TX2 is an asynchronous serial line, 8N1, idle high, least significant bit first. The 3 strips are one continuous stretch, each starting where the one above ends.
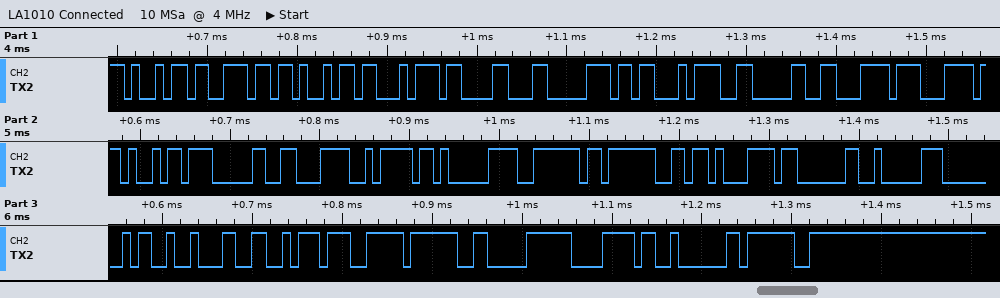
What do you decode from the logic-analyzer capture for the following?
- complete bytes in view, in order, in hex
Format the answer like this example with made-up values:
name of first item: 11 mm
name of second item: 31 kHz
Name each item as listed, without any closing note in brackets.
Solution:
complete bytes in view, in order, in hex: 0x69 0x6E 0x69 0x74 0x18 0x70 0xA3 0x06 0xC6 0xC7 0x4B 0x07 0xC6 0x7A 0xC1 0x7E 0x3F 0x8B 0x03 0x82 0x40 0x12 0xA6 0xE7 0x3F 0xF0 0x78 0x02 0x3F
